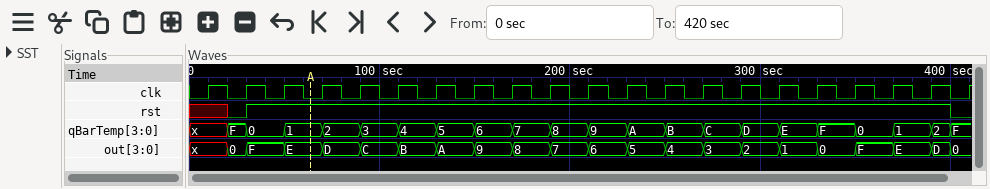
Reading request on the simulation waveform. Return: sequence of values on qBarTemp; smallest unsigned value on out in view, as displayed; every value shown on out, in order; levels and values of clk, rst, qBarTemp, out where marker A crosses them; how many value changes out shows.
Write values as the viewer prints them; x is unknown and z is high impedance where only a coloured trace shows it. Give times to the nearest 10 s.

x, F, 0, 1, 2, 3, 4, 5, 6, 7, 8, 9, A, B, C, D, E, F, 0, 1, 2, F
0
x, 0, F, E, D, C, B, A, 9, 8, 7, 6, 5, 4, 3, 2, 1, 0, F, E, D, 0
clk=0, rst=1, qBarTemp=1, out=E
21
